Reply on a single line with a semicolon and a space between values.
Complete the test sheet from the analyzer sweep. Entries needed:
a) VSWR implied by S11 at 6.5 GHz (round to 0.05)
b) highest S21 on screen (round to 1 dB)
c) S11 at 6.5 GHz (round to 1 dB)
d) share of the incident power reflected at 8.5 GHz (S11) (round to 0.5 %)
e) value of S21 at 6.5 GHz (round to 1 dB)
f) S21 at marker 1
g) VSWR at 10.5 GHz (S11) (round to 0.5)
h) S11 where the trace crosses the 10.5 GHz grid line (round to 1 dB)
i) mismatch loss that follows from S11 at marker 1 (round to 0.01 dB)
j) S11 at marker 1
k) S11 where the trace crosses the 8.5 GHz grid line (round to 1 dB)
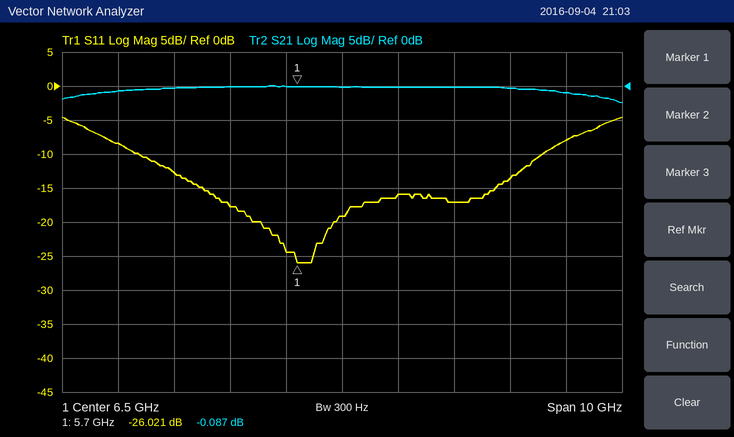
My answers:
1.25; 0 dB; -19 dB; 2.0 %; 0 dB; -0.087 dB; 2.5; -8 dB; 0.01 dB; -26.021 dB; -17 dB
